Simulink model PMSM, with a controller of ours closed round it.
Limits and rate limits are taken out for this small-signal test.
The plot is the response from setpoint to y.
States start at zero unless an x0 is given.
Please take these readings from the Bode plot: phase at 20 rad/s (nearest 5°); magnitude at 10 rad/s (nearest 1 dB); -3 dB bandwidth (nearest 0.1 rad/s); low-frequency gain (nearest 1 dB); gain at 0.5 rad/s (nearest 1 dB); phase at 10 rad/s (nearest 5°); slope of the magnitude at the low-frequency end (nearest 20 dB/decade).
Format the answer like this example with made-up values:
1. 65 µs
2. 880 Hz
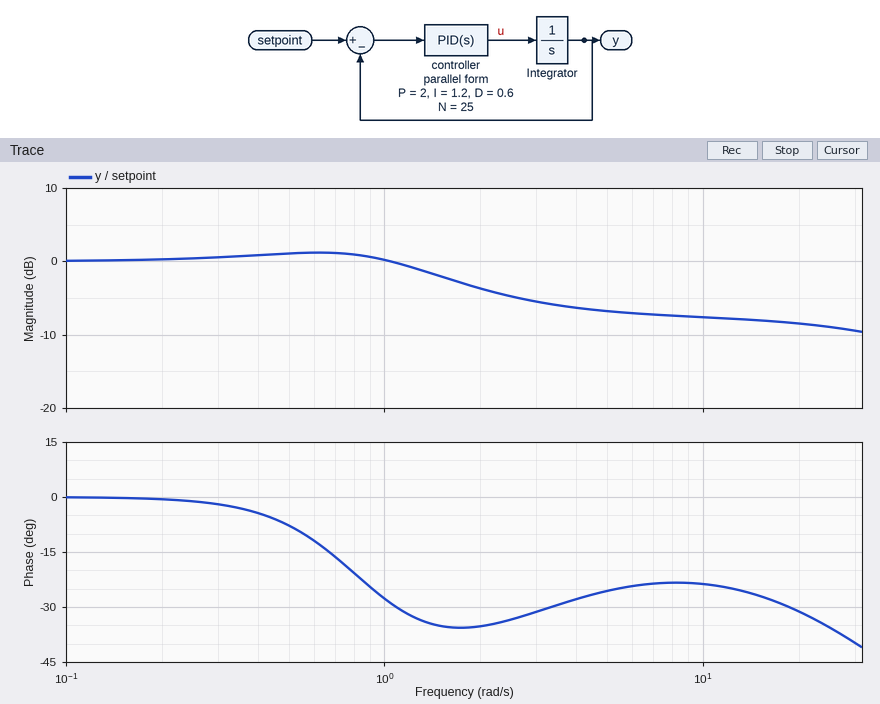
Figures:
1. -30°
2. -8 dB
3. 1.7 rad/s
4. 0 dB
5. 1 dB
6. -25°
7. 0 dB/decade
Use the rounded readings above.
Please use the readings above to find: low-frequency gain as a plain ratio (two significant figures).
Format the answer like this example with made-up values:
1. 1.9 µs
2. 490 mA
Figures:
1. 1.0
